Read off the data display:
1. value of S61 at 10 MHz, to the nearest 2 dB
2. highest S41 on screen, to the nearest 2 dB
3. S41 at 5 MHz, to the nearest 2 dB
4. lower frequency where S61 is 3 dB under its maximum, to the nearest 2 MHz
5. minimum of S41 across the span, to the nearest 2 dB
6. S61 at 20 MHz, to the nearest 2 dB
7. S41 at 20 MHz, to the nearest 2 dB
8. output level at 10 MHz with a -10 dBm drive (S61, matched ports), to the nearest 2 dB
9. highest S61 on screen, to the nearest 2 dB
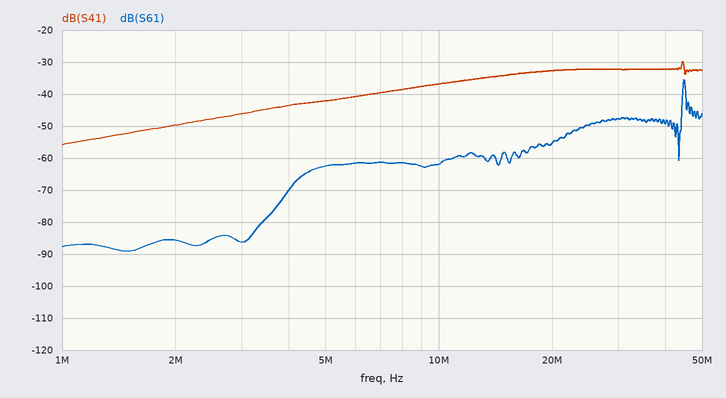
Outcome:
-62 dB
-30 dB
-42 dB
44 MHz
-56 dB
-56 dB
-32 dB
-72 dBm
-36 dB
